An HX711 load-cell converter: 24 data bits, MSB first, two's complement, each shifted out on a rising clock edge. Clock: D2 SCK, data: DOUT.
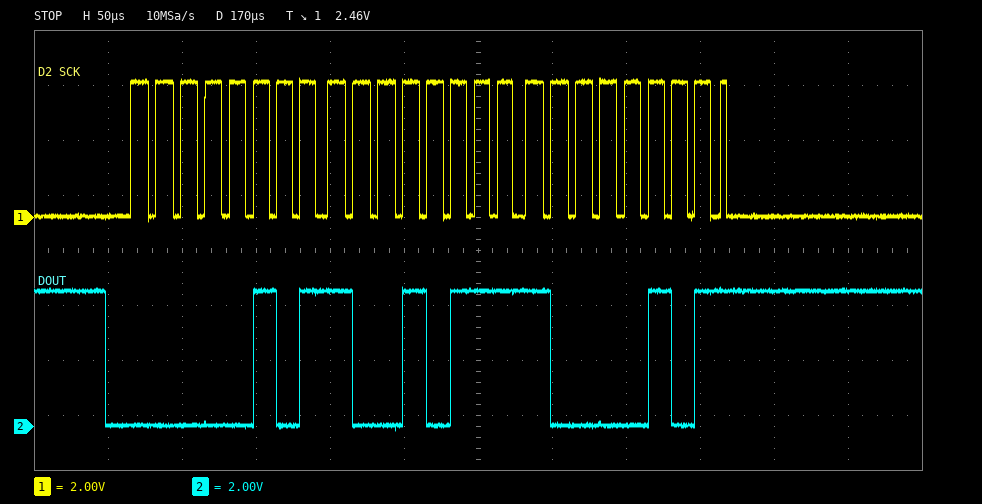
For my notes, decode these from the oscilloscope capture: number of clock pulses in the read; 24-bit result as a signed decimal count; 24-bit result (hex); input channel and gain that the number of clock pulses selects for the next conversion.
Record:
25
366469
0x059785
channel A, gain 128
